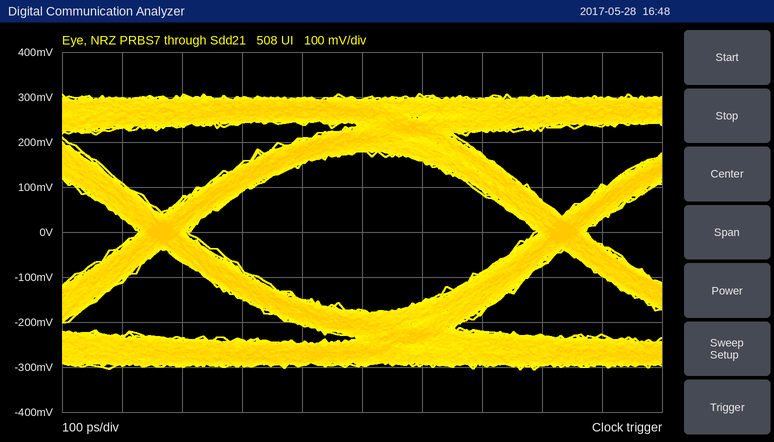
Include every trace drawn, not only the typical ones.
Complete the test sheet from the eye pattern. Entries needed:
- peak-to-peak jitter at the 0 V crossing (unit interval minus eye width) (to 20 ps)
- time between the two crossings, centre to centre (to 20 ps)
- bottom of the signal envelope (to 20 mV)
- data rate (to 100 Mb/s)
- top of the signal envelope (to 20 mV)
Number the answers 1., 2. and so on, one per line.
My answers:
1. 80 ps
2. 660 ps
3. -300 mV
4. 1.5 Gb/s
5. 300 mV
